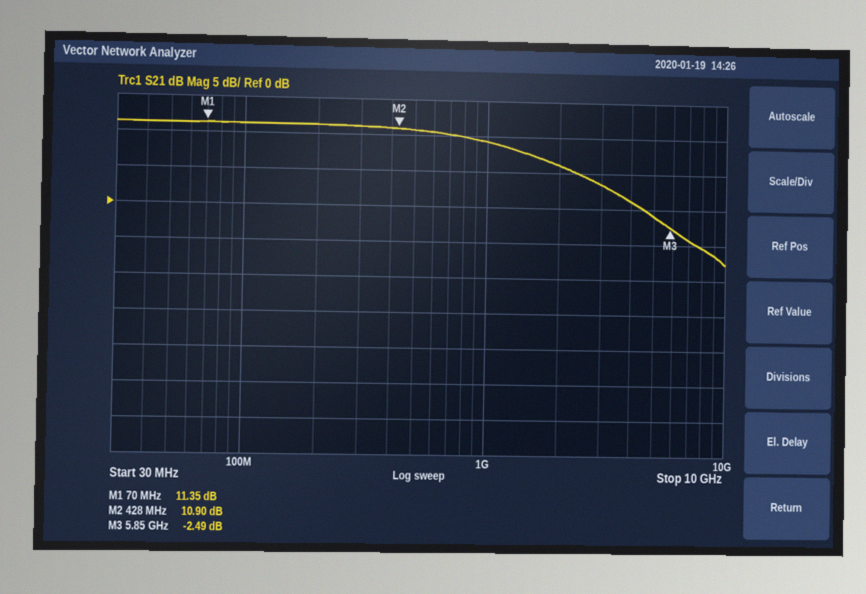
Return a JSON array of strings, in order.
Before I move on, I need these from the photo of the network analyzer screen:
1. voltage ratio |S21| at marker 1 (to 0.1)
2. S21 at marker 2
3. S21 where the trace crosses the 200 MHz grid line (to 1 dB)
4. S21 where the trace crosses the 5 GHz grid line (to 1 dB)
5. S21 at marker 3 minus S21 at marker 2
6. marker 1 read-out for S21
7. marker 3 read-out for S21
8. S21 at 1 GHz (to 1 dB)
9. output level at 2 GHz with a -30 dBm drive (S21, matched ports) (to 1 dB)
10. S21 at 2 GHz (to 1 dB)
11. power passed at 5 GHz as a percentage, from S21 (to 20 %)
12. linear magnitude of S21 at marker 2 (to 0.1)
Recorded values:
["3.7", "10.90 dB", "11 dB", "-1 dB", "-13.39 dB", "11.35 dB", "-2.49 dB", "9 dB", "-24 dBm", "6 dB", "80 %", "3.5"]
